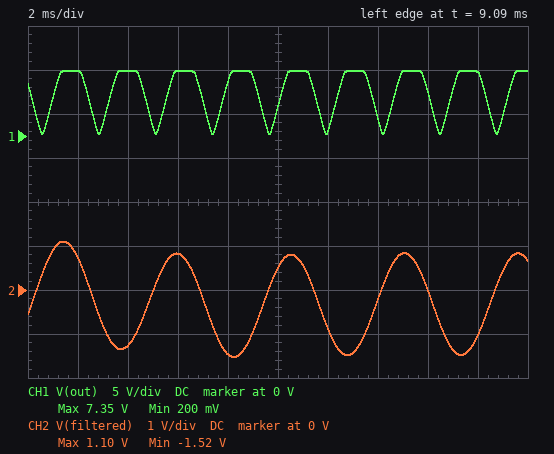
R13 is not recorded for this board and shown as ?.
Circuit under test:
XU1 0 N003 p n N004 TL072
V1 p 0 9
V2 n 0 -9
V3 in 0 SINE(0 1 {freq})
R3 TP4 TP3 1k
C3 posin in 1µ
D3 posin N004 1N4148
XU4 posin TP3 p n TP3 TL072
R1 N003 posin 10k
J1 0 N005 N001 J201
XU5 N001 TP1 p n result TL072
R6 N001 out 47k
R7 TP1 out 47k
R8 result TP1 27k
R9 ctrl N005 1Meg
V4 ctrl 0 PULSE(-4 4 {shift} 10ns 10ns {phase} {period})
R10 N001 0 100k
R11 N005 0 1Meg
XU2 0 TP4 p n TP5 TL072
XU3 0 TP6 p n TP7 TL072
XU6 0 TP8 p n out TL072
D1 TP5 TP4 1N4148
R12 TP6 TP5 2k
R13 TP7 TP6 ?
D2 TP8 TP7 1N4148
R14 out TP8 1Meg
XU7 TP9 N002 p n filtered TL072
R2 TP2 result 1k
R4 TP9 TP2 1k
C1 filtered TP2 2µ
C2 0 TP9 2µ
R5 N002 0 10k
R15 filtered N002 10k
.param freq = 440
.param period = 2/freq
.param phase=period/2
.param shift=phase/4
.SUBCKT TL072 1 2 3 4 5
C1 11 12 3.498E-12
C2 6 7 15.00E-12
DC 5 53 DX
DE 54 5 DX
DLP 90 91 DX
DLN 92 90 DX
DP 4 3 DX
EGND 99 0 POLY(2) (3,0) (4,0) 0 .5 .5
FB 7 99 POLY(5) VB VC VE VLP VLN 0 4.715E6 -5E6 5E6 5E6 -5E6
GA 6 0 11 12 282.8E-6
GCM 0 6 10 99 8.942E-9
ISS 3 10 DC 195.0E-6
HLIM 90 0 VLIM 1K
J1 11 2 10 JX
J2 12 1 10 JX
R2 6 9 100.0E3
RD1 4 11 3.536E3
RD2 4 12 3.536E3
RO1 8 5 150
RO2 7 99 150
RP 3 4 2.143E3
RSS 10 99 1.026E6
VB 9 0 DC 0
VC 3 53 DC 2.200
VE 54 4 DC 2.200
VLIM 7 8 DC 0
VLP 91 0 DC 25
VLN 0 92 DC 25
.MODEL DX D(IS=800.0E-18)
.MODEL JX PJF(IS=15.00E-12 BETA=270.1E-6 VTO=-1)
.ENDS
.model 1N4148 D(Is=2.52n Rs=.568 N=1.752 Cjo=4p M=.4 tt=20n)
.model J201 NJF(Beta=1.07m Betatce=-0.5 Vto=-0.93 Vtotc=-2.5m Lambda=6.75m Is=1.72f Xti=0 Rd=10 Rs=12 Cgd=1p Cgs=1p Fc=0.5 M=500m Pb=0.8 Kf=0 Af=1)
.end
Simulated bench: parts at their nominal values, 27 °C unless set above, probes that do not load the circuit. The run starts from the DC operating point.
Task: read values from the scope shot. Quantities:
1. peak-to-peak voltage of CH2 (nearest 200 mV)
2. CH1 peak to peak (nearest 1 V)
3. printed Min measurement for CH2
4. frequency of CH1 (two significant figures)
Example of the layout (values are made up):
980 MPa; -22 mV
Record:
2.6 V; 7 V; -1.52 V; 440 Hz
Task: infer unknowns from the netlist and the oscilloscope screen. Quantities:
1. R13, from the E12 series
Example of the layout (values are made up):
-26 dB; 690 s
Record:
1.2 kΩ
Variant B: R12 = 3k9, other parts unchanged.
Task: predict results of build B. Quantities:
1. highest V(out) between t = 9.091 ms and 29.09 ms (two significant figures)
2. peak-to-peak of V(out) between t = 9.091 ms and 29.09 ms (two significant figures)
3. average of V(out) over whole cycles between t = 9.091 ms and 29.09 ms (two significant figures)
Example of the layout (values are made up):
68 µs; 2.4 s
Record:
160 mV; 140 mV; 120 mV
